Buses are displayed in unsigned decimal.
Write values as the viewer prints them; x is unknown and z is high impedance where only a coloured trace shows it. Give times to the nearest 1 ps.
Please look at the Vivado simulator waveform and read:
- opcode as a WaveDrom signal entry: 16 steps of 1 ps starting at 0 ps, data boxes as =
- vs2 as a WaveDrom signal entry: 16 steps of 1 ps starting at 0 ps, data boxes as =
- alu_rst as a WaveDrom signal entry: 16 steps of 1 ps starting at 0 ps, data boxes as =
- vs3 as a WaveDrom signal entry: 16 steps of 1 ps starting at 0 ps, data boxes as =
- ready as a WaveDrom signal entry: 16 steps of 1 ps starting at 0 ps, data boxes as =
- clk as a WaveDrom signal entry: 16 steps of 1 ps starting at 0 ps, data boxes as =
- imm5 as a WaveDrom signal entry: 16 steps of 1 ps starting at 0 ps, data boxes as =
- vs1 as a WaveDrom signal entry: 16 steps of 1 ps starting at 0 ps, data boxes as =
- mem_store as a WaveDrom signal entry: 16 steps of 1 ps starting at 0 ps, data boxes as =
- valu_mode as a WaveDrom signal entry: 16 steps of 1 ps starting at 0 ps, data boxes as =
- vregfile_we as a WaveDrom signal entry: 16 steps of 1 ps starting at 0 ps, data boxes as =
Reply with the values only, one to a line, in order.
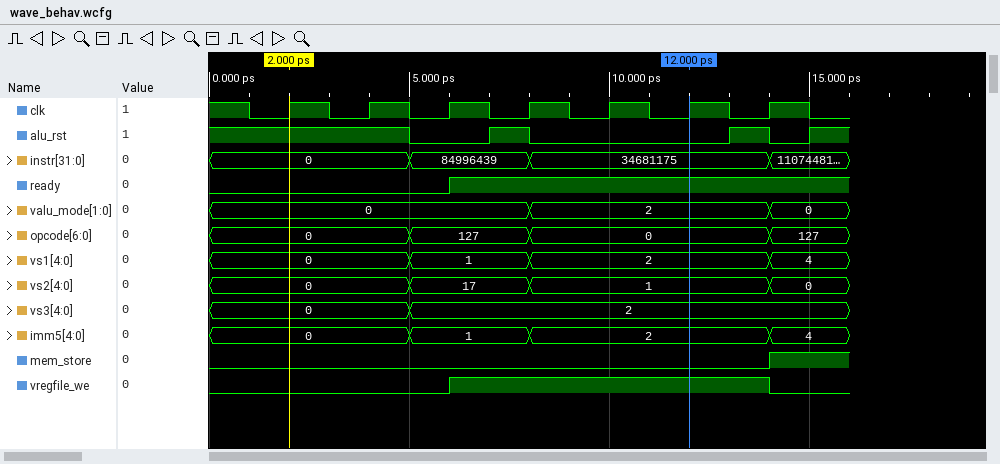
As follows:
{name: 'opcode', wave: '=....=..=.....=.', data: '0 127 0 127'}
{name: 'vs2', wave: '=....=..=.....=.', data: '0 17 1 0'}
{name: 'alu_rst', wave: '1....0.10....101'}
{name: 'vs3', wave: '=....=..........', data: '0 2'}
{name: 'ready', wave: '0.....1.........'}
{name: 'clk', wave: '1010101010101010'}
{name: 'imm5', wave: '=....=..=.....=.', data: '0 1 2 4'}
{name: 'vs1', wave: '=....=..=.....=.', data: '0 1 2 4'}
{name: 'mem_store', wave: '0.............1.'}
{name: 'valu_mode', wave: '=.......=.....=.', data: '0 2 0'}
{name: 'vregfile_we', wave: '0.....1.......0.'}
